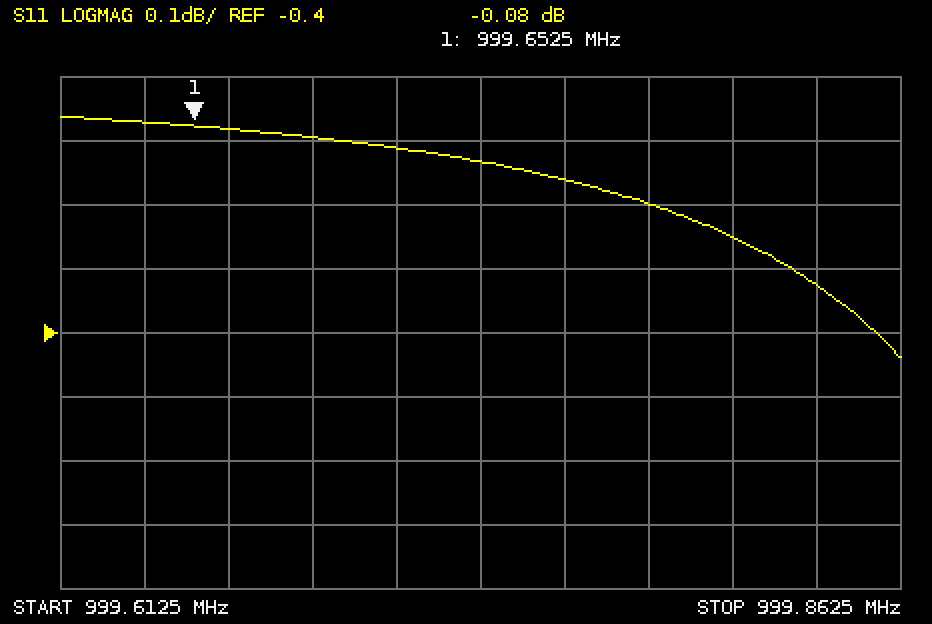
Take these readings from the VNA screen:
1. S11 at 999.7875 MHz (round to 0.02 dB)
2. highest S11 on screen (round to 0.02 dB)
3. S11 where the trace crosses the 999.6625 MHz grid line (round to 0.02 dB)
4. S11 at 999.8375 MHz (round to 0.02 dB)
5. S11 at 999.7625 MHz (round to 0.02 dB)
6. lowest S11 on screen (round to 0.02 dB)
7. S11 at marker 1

-0.20 dB
-0.06 dB
-0.08 dB
-0.32 dB
-0.16 dB
-0.44 dB
-0.08 dB
